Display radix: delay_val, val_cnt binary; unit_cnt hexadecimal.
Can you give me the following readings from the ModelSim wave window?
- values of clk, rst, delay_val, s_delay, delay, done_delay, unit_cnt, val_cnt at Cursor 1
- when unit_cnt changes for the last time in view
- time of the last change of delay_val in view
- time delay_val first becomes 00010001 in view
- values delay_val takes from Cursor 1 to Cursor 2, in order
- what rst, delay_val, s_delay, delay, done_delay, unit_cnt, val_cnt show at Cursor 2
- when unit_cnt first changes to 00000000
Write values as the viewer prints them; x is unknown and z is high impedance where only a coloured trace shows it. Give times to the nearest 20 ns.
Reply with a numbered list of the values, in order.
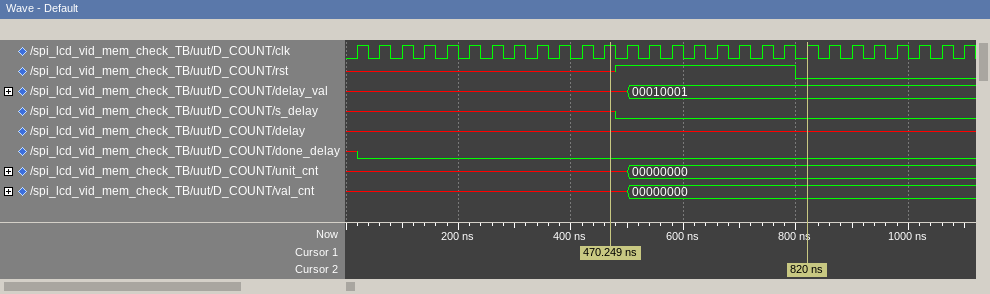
1. clk=1, rst=x, delay_val=x, s_delay=x, delay=x, done_delay=0, unit_cnt=x, val_cnt=x
2. 500 ns
3. 500 ns
4. 500 ns
5. x, 00010001
6. rst=0, delay_val=00010001, s_delay=0, delay=x, done_delay=0, unit_cnt=00000000, val_cnt=00000000
7. 500 ns
